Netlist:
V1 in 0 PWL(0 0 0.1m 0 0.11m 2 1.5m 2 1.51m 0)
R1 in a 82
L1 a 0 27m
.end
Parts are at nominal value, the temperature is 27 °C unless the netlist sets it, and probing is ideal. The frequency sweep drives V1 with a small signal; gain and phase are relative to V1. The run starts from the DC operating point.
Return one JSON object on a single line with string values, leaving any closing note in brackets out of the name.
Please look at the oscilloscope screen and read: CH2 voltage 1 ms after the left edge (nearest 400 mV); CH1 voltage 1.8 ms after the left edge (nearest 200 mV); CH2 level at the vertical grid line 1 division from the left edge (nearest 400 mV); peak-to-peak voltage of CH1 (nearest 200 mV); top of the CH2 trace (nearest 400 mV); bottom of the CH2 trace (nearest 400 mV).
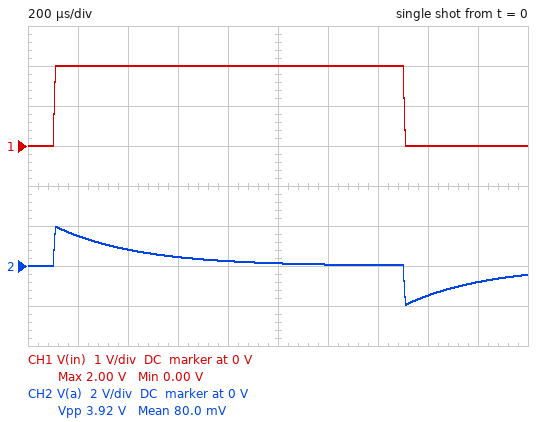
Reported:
{"CH2 voltage 1 ms after the left edge": "0 V", "CH1 voltage 1.8 ms after the left edge": "0 V", "CH2 level at the vertical grid line 1 division from the left edge": "1.6 V", "peak-to-peak voltage of CH1": "2.0 V", "top of the CH2 trace": "2.0 V", "bottom of the CH2 trace": "-2.0 V"}
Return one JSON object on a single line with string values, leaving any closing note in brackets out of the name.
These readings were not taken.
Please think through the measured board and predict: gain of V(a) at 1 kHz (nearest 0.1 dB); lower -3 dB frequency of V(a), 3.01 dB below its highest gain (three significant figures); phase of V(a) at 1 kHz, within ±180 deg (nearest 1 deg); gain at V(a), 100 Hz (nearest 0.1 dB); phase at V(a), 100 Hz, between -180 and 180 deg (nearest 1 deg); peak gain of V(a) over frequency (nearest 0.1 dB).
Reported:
{"gain of V(a) at 1 kHz": "-0.9 dB", "lower -3 dB frequency of V(a), 3.01 dB below its highest gain": "483 Hz", "phase of V(a) at 1 kHz, within ±180 deg": "26 deg", "gain at V(a), 100 Hz": "-13.9 dB", "phase at V(a), 100 Hz, between -180 and 180 deg": "78 deg", "peak gain of V(a) over frequency": "0 dB"}
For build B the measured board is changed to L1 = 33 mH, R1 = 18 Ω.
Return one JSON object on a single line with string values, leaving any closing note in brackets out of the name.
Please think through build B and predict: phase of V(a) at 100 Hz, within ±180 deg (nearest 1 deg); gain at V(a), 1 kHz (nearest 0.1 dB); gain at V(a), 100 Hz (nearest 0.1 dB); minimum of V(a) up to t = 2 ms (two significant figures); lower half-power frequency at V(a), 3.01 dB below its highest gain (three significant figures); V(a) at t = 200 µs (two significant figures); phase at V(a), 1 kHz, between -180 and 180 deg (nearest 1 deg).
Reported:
{"phase of V(a) at 100 Hz, within ±180 deg": "41 deg", "gain at V(a), 1 kHz": "0 dB", "gain at V(a), 100 Hz": "-2.4 dB", "minimum of V(a) up to t = 2 ms": "-1.1 V", "lower half-power frequency at V(a), 3.01 dB below its highest gain": "86.8 Hz", "V(a) at t = 200 µs": "1.9 V", "phase at V(a), 1 kHz, between -180 and 180 deg": "5 deg"}
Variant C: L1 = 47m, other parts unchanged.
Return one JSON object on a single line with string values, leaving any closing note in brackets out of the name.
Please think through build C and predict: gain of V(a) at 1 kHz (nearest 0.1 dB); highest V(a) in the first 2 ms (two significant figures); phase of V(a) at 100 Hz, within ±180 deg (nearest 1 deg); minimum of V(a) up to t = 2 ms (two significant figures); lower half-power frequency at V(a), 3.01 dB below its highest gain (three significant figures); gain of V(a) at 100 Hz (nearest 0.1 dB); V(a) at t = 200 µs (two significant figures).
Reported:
{"gain of V(a) at 1 kHz": "-0.3 dB", "highest V(a) in the first 2 ms": "2.0 V", "phase of V(a) at 100 Hz, within ±180 deg": "70 deg", "minimum of V(a) up to t = 2 ms": "-1.8 V", "lower half-power frequency at V(a), 3.01 dB below its highest gain": "278 Hz", "gain of V(a) at 100 Hz": "-9.4 dB", "V(a) at t = 200 µs": "1.7 V"}
